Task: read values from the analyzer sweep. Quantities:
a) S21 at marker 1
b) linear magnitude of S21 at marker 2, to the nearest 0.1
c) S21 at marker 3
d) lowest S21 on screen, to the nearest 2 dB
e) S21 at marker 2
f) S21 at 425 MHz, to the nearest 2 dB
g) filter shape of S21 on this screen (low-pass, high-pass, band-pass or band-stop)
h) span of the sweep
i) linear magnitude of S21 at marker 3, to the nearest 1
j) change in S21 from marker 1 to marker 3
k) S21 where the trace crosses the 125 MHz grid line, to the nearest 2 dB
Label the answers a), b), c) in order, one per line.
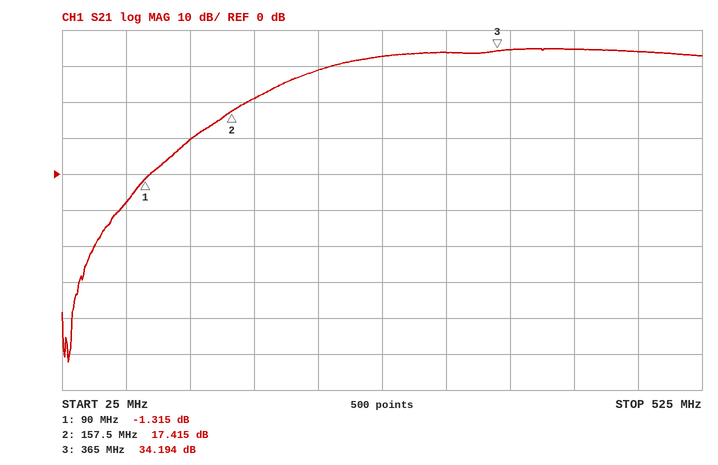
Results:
a) -1.315 dB
b) 7.4
c) 34.194 dB
d) -52 dB
e) 17.415 dB
f) 34 dB
g) high-pass
h) 500 MHz
i) 51
j) 35.509 dB
k) 10 dB
